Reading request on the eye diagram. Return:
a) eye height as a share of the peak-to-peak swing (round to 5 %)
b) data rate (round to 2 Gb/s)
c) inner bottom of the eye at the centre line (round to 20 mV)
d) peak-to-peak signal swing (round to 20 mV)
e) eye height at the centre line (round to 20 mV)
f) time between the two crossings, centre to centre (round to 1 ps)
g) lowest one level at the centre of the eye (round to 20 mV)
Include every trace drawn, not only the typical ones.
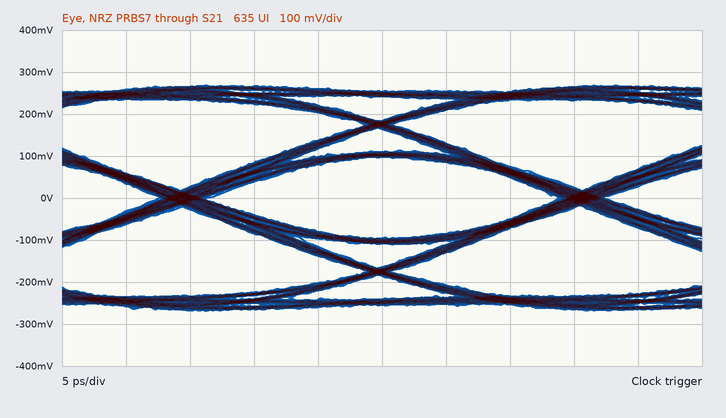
35 %
32 Gb/s
-100 mV
540 mV
200 mV
31 ps
100 mV
